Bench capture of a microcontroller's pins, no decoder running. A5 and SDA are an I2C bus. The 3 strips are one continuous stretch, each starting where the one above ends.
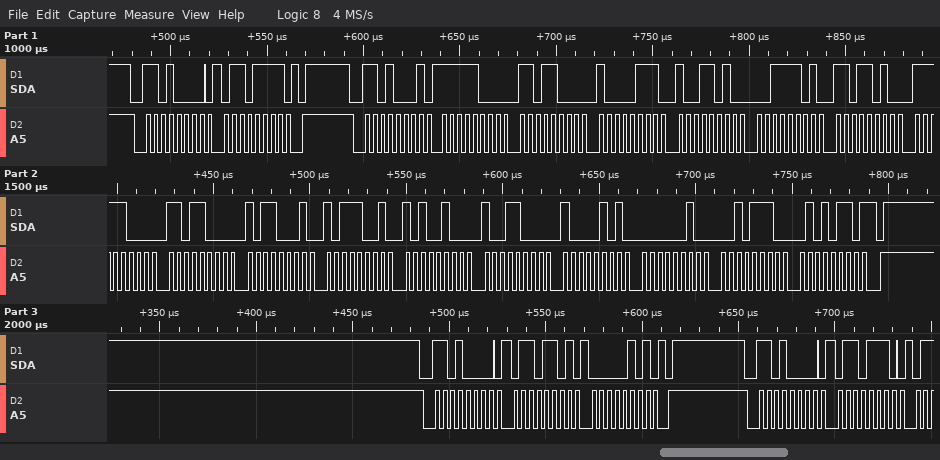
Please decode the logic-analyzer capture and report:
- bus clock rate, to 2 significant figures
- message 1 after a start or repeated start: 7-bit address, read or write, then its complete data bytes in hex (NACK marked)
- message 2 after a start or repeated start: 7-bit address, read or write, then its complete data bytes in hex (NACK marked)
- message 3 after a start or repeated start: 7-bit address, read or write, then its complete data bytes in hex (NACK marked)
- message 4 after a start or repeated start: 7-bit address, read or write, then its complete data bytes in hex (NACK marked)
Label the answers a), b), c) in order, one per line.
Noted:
a) 250 kHz
b) 0x68 write: 6F
c) 0x68 read: F8 D8 87 9A 3D DA F8 D8 B1 B9 A4 98 85 02 2E 56 NACK
d) 0x68 write: 6D 05
e) 0x68 write: 6E
